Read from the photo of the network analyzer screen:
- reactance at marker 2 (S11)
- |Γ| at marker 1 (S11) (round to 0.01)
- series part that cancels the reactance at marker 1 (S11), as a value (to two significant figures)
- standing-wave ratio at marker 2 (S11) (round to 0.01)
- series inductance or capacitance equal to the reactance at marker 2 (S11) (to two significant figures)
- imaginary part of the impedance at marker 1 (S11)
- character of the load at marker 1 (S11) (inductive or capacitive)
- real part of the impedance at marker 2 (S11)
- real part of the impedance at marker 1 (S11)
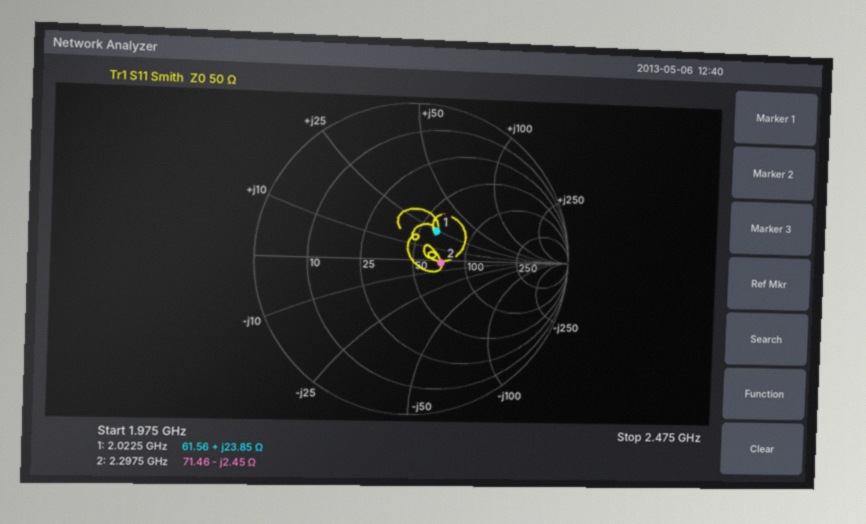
-2.45 Ω
0.23
3.3 pF
1.43
28 pF
+23.85 Ω
inductive
71.46 Ω
61.56 Ω
